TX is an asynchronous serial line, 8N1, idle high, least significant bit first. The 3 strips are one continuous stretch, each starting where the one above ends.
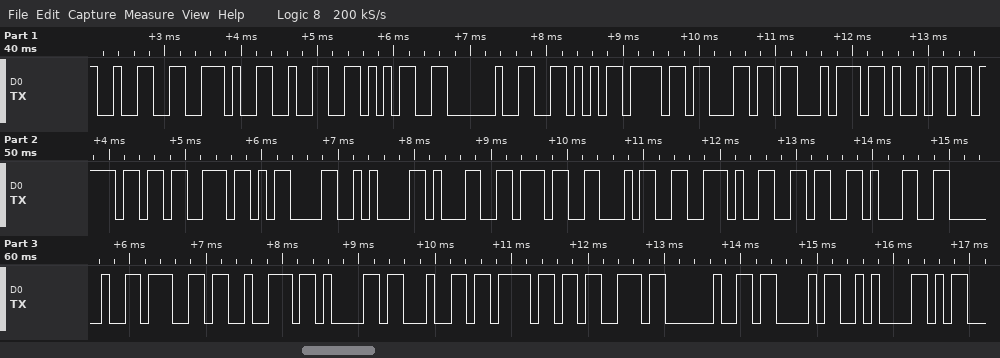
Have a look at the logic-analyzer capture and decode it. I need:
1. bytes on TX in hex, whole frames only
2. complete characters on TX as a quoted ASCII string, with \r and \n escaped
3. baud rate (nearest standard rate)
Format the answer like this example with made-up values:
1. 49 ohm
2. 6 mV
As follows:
1. 32 2E 32 35 20 56 6F 6C 74 69 6F 73 0D 0A 31 37 34 2E 36 31 20 67 72 61 64 6F 73 20 43 0A
2. "2.25 Voltios\r\n174.61 grados C\n"
3. 9600 baud
